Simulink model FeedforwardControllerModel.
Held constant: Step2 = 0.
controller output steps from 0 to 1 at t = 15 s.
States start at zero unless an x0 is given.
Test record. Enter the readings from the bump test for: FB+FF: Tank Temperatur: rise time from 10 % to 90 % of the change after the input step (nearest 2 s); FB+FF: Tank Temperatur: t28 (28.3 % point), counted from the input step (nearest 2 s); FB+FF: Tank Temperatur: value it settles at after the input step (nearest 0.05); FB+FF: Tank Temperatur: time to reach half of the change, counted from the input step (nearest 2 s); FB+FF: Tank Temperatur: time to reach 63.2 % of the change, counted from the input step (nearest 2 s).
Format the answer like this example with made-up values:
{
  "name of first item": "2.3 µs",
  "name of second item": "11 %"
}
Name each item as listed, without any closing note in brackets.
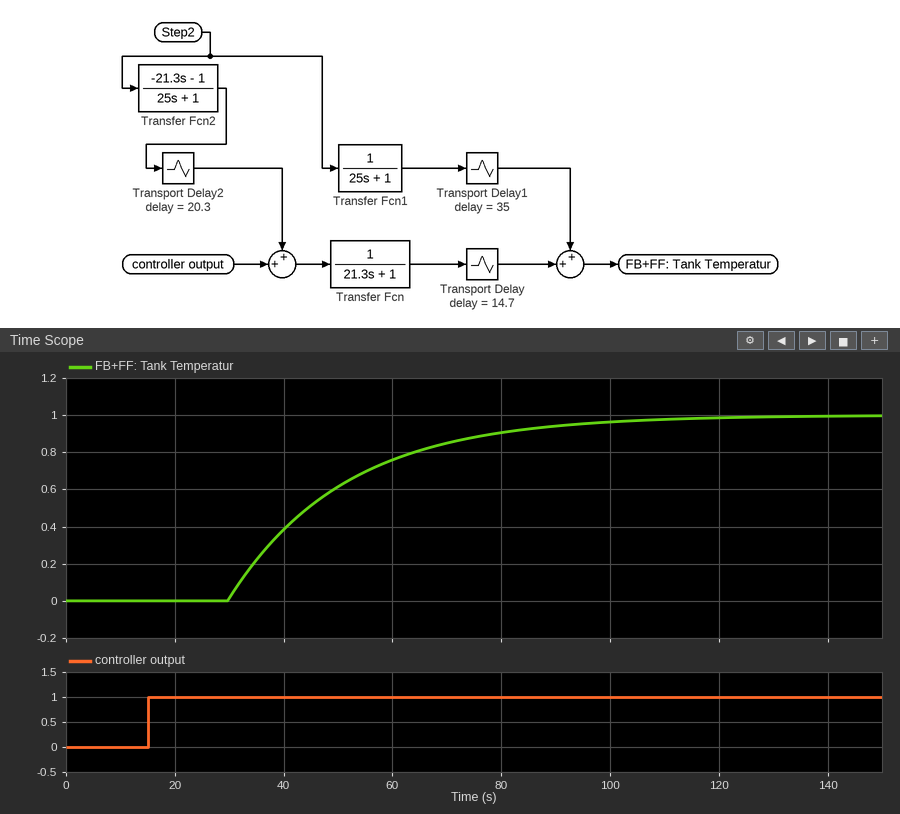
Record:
{
  "FB+FF: Tank Temperatur: rise time from 10 % to 90 % of the change after the input step": "46 s",
  "FB+FF: Tank Temperatur: t28 (28.3 % point), counted from the input step": "22 s",
  "FB+FF: Tank Temperatur: value it settles at after the input step": "1.00",
  "FB+FF: Tank Temperatur: time to reach half of the change, counted from the input step": "30 s",
  "FB+FF: Tank Temperatur: time to reach 63.2 % of the change, counted from the input step": "36 s"
}
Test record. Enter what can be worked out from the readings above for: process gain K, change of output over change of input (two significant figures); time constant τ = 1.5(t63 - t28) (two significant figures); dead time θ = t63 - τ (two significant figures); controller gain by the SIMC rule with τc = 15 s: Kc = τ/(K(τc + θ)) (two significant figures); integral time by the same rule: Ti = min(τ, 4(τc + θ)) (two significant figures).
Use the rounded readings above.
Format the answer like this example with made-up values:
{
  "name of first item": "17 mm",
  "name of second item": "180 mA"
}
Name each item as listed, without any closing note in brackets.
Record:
{
  "process gain K, change of output over change of input": "1.0",
  "time constant τ = 1.5(t63 - t28)": "21 s",
  "dead time θ = t63 - τ": "15 s",
  "controller gain by the SIMC rule with τc = 15 s: Kc = τ/(K(τc + θ))": "0.70",
  "integral time by the same rule: Ti = min(τ, 4(τc + θ))": "21 s"
}
